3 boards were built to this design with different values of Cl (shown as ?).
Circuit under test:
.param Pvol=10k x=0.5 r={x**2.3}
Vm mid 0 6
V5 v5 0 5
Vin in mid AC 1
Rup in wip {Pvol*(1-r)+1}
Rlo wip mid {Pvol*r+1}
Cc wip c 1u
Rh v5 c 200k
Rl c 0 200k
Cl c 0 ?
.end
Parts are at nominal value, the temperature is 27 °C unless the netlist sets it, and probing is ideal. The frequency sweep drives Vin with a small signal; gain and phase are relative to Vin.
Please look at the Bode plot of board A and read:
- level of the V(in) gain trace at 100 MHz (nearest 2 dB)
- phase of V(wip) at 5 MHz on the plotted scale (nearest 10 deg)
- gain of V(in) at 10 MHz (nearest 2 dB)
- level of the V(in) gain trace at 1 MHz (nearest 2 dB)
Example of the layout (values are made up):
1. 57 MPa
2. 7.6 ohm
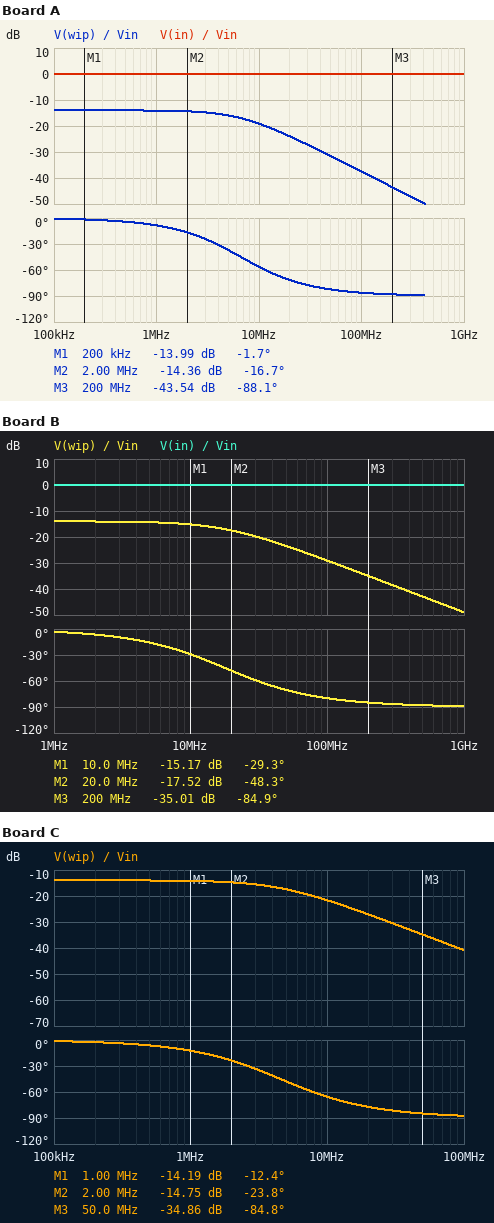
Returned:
1. 0 dB
2. -40 deg
3. 0 dB
4. 0 dB
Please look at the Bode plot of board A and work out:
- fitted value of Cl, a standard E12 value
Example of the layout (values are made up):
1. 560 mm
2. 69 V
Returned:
1. 15 pF
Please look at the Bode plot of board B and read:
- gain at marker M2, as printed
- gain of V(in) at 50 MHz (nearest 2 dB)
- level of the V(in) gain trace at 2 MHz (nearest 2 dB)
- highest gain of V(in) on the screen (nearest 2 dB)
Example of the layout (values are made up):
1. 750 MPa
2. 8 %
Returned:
1. -17.52 dB
2. 0 dB
3. 0 dB
4. 0 dB
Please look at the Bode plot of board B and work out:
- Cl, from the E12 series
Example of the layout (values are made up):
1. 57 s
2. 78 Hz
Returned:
1. 5.6 pF
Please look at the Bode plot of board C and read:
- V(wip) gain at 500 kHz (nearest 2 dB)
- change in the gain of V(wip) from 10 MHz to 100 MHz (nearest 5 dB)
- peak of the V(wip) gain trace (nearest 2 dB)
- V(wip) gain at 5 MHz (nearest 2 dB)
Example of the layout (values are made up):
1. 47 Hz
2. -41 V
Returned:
1. -14 dB
2. -20 dB
3. -14 dB
4. -18 dB
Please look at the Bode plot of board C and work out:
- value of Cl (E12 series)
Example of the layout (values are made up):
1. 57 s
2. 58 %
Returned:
1. 22 pF
